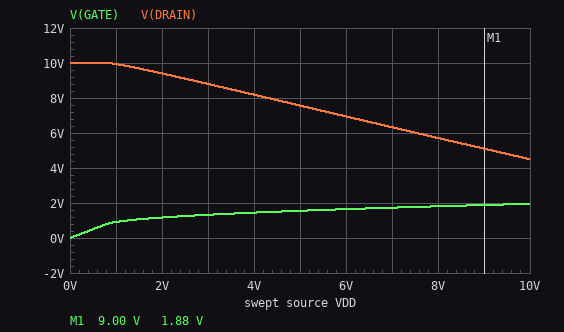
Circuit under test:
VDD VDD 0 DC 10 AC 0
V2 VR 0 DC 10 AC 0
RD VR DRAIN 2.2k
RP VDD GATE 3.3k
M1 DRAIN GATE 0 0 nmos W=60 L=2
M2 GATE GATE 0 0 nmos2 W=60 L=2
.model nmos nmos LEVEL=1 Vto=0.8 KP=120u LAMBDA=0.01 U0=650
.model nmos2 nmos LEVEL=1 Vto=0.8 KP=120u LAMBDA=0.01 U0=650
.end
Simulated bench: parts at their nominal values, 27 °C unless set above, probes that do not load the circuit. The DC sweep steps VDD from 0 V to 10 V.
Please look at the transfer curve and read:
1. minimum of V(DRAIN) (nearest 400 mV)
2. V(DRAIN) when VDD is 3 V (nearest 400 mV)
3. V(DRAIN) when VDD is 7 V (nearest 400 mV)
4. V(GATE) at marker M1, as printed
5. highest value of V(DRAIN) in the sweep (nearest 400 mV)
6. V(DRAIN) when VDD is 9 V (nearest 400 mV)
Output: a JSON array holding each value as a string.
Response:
["4.4 V", "8.8 V", "6.4 V", "1.88 V", "10.0 V", "5.2 V"]
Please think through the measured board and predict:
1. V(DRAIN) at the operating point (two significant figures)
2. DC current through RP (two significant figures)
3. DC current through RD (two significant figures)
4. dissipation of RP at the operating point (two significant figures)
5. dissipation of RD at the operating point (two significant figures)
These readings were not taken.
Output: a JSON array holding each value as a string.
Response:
["4.5 V", "2.4 mA", "2.5 mA", "20 mW", "14 mW"]
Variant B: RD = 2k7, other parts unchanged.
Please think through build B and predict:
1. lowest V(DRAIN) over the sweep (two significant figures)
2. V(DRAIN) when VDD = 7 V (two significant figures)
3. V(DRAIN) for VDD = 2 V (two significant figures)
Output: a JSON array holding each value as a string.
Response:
["3.3 V", "5.5 V", "9.3 V"]
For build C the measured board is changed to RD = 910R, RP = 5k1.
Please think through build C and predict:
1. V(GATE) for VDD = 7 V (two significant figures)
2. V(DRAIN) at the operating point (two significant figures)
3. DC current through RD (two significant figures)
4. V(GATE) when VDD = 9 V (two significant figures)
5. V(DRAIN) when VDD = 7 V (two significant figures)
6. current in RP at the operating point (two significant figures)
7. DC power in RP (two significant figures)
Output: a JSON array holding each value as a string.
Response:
["1.6 V", "8.4 V", "1.7 mA", "1.7 V", "9.0 V", "1.6 mA", "13 mW"]
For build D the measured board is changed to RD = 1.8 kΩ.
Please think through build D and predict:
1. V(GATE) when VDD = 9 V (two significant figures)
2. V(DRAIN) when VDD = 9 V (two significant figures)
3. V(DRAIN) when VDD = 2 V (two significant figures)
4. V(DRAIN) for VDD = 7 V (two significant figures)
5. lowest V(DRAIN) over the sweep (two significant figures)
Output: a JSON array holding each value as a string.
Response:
["1.9 V", "6.0 V", "9.5 V", "7.0 V", "5.5 V"]
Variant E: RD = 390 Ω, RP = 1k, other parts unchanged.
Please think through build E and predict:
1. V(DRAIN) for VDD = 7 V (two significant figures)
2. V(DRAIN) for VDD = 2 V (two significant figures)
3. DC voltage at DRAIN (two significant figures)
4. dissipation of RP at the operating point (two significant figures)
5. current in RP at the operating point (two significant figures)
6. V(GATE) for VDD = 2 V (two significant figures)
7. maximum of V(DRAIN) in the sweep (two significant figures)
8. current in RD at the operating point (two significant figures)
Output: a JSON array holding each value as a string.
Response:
["8.1 V", "9.7 V", "7.1 V", "52 mW", "7.2 mA", "1.4 V", "10 V", "7.5 mA"]
